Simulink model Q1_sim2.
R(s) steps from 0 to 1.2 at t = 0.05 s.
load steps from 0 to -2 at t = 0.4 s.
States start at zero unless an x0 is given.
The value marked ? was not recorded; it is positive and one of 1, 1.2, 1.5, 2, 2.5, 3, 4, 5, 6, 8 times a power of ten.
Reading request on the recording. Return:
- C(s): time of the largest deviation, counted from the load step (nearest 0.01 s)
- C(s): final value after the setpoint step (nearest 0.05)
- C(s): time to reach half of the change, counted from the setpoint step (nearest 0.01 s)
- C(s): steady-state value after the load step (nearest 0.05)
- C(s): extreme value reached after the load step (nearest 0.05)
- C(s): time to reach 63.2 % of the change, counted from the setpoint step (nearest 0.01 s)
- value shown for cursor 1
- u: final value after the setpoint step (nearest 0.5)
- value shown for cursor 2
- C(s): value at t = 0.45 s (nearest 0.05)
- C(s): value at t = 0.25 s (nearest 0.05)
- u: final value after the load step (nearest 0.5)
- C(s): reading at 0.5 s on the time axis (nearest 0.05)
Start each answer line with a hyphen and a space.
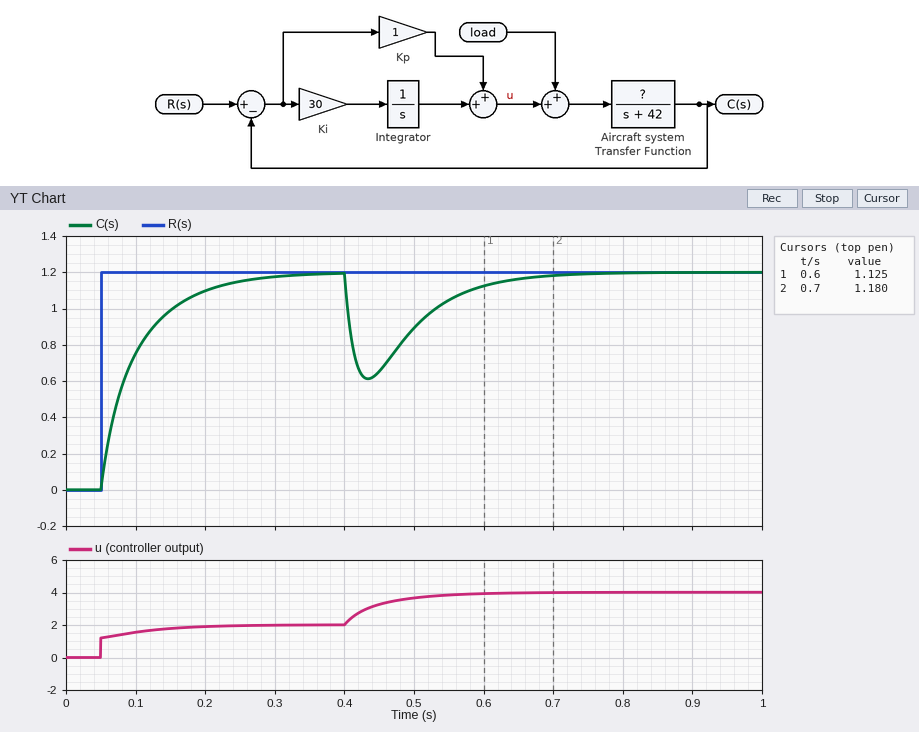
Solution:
- 0.03 s
- 1.20
- 0.03 s
- 1.20
- 0.60
- 0.05 s
- 1.125
- 2.0
- 1.180
- 0.65
- 1.15
- 4.0
- 0.90
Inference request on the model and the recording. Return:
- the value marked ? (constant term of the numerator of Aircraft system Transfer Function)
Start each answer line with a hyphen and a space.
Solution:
- 25
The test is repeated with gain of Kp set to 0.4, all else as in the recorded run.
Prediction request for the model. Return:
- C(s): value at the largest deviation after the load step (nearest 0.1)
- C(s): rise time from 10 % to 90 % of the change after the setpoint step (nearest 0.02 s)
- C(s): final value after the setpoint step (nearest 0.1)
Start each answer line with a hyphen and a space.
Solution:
- 0.5
- 0.10 s
- 1.2
